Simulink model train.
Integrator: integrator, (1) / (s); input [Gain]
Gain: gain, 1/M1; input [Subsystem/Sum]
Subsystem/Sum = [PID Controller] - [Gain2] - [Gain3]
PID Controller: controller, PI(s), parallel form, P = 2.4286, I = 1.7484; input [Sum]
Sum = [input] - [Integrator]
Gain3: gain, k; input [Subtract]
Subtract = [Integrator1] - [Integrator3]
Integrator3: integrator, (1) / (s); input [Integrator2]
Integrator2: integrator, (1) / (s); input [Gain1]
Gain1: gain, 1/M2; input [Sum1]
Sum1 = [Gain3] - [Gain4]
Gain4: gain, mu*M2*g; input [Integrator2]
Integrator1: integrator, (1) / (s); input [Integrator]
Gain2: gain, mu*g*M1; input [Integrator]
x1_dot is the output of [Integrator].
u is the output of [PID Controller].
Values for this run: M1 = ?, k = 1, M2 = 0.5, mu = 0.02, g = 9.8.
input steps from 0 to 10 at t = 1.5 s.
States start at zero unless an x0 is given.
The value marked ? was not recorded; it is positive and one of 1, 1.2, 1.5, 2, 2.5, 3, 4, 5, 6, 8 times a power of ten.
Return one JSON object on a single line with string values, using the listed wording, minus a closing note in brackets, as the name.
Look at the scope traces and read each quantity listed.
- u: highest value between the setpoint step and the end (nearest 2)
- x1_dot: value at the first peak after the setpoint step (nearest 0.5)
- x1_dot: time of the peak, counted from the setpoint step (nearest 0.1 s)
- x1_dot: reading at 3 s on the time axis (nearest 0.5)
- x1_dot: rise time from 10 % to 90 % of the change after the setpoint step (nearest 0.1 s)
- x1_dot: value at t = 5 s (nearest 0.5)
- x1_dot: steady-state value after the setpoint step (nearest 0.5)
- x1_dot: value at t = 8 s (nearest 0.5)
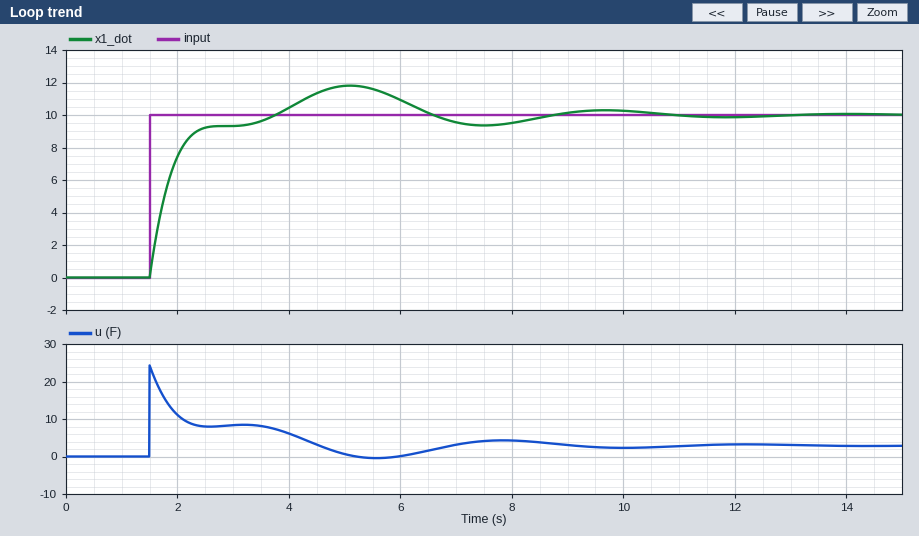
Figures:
{"u: highest value between the setpoint step and the end": "24", "x1_dot: value at the first peak after the setpoint step": "12.0", "x1_dot: time of the peak, counted from the setpoint step": "3.6 s", "x1_dot: reading at 3 s on the time axis": "9.5", "x1_dot: rise time from 10 % to 90 % of the change after the setpoint step": "0.8 s", "x1_dot: value at t = 5 s": "12.0", "x1_dot: steady-state value after the setpoint step": "10.0", "x1_dot: value at t = 8 s": "9.5"}
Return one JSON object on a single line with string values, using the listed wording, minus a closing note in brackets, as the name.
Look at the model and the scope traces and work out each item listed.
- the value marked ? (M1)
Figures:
{"the value marked ?": "1"}
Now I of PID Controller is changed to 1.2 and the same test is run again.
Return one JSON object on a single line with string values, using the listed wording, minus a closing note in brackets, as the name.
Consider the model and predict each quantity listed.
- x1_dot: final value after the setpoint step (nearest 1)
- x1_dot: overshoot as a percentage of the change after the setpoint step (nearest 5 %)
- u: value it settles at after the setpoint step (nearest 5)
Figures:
{"x1_dot: final value after the setpoint step": "10", "x1_dot: overshoot as a percentage of the change after the setpoint step": "15 %", "u: value it settles at after the setpoint step": "5"}
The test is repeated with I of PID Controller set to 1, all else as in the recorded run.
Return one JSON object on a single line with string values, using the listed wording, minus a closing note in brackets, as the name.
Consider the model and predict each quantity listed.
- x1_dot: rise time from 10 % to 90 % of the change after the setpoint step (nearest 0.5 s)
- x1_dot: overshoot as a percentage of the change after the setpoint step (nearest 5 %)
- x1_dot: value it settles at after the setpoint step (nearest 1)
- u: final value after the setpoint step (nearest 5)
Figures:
{"x1_dot: rise time from 10 % to 90 % of the change after the setpoint step": "2.0 s", "x1_dot: overshoot as a percentage of the change after the setpoint step": "15 %", "x1_dot: value it settles at after the setpoint step": "10", "u: final value after the setpoint step": "5"}
